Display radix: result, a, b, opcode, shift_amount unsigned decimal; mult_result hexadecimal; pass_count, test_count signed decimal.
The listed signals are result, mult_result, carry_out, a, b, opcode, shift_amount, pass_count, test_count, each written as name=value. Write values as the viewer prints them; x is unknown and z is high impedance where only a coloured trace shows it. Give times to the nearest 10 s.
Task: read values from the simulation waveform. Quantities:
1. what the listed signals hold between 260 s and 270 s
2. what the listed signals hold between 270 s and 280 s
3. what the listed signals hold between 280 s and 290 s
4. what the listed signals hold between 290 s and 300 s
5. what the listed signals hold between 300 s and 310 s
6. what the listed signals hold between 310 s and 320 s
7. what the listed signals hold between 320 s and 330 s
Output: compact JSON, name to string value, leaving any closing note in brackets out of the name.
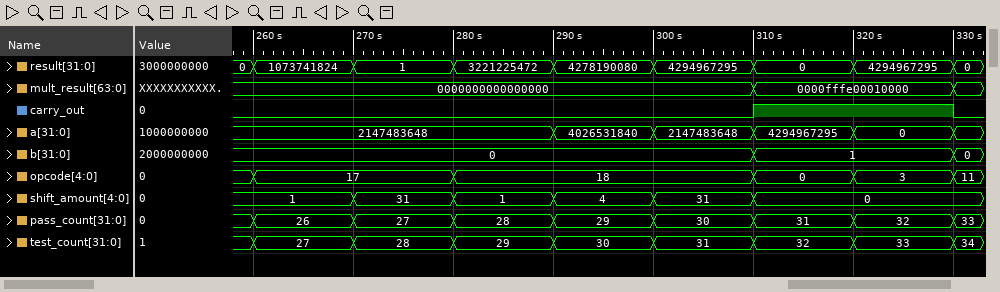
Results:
{"what the listed signals hold between 260 s and 270 s": "result=1073741824, mult_result=0000000000000000, carry_out=0, a=2147483648, b=0, opcode=17, shift_amount=1, pass_count=26, test_count=27", "what the listed signals hold between 270 s and 280 s": "result=1, mult_result=0000000000000000, carry_out=0, a=2147483648, b=0, opcode=17, shift_amount=31, pass_count=27, test_count=28", "what the listed signals hold between 280 s and 290 s": "result=3221225472, mult_result=0000000000000000, carry_out=0, a=2147483648, b=0, opcode=18, shift_amount=1, pass_count=28, test_count=29", "what the listed signals hold between 290 s and 300 s": "result=4278190080, mult_result=0000000000000000, carry_out=0, a=4026531840, b=0, opcode=18, shift_amount=4, pass_count=29, test_count=30", "what the listed signals hold between 300 s and 310 s": "result=4294967295, mult_result=0000000000000000, carry_out=0, a=2147483648, b=0, opcode=18, shift_amount=31, pass_count=30, test_count=31", "what the listed signals hold between 310 s and 320 s": "result=0, mult_result=0000fffe00010000, carry_out=1, a=4294967295, b=1, opcode=0, shift_amount=0, pass_count=31, test_count=32", "what the listed signals hold between 320 s and 330 s": "result=4294967295, mult_result=0000fffe00010000, carry_out=1, a=0, b=1, opcode=3, shift_amount=0, pass_count=32, test_count=33"}
